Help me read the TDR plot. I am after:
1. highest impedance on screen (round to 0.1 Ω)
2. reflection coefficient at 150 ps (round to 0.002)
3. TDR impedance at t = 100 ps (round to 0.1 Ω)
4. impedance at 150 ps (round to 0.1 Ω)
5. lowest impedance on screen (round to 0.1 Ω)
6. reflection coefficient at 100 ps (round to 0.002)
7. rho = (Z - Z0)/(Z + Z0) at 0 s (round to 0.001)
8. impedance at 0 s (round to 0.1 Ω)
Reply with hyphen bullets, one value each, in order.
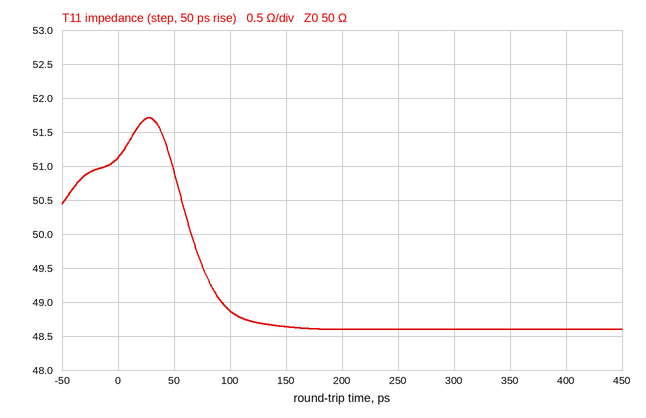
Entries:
- 51.7 Ω
- -0.014
- 48.9 Ω
- 48.6 Ω
- 48.6 Ω
- -0.012
- +0.011
- 51.1 Ω
